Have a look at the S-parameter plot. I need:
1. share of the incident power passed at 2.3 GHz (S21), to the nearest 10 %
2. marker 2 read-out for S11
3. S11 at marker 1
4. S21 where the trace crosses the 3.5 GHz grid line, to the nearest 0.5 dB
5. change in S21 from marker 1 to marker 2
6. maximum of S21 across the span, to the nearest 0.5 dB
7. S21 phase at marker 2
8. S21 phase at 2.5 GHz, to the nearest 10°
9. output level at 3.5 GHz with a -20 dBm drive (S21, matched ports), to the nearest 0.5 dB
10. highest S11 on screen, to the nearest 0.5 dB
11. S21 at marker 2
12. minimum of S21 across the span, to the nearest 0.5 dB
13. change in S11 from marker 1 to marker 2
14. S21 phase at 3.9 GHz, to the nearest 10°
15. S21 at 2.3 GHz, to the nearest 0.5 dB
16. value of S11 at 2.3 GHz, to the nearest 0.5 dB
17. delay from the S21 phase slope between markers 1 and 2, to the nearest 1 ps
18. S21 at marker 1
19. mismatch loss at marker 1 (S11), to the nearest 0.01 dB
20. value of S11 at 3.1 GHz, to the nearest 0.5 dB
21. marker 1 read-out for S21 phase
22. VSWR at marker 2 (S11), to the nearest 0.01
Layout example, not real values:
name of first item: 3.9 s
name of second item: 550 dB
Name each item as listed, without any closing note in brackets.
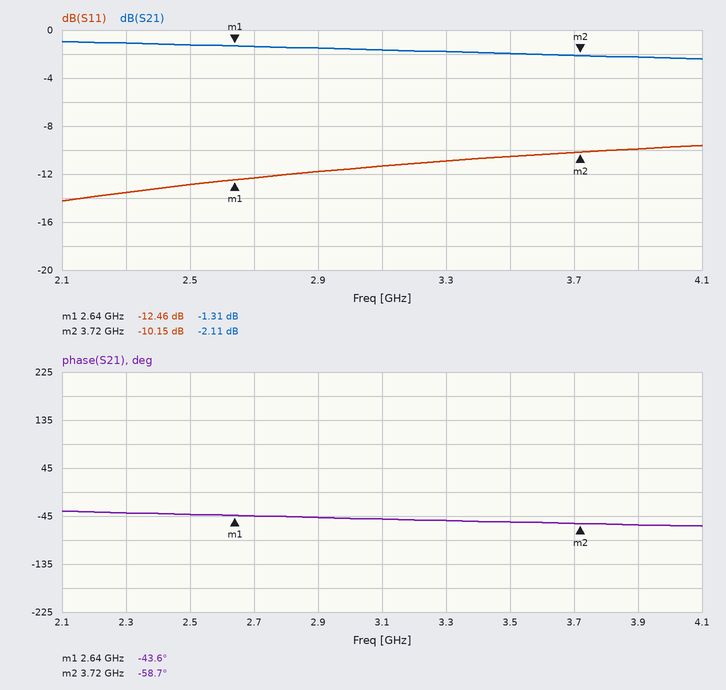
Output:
share of the incident power passed at 2.3 GHz (S21), to the nearest 10 %: 80 %
marker 2 read-out for S11: -10.15 dB
S11 at marker 1: -12.46 dB
S21 where the trace crosses the 3.5 GHz grid line, to the nearest 0.5 dB: -2.0 dB
change in S21 from marker 1 to marker 2: -0.80 dB
maximum of S21 across the span, to the nearest 0.5 dB: -1.0 dB
S21 phase at marker 2: -58.7°
S21 phase at 2.5 GHz, to the nearest 10°: -40°
output level at 3.5 GHz with a -20 dBm drive (S21, matched ports), to the nearest 0.5 dB: -22.0 dBm
highest S11 on screen, to the nearest 0.5 dB: -9.5 dB
S21 at marker 2: -2.11 dB
minimum of S21 across the span, to the nearest 0.5 dB: -2.5 dB
change in S11 from marker 1 to marker 2: 2.31 dB
S21 phase at 3.9 GHz, to the nearest 10°: -60°
S21 at 2.3 GHz, to the nearest 0.5 dB: -1.0 dB
value of S11 at 2.3 GHz, to the nearest 0.5 dB: -13.5 dB
delay from the S21 phase slope between markers 1 and 2, to the nearest 1 ps: 39 ps
S21 at marker 1: -1.31 dB
mismatch loss at marker 1 (S11), to the nearest 0.01 dB: 0.25 dB
value of S11 at 3.1 GHz, to the nearest 0.5 dB: -11.5 dB
marker 1 read-out for S21 phase: -43.6°
VSWR at marker 2 (S11), to the nearest 0.01: 1.90
